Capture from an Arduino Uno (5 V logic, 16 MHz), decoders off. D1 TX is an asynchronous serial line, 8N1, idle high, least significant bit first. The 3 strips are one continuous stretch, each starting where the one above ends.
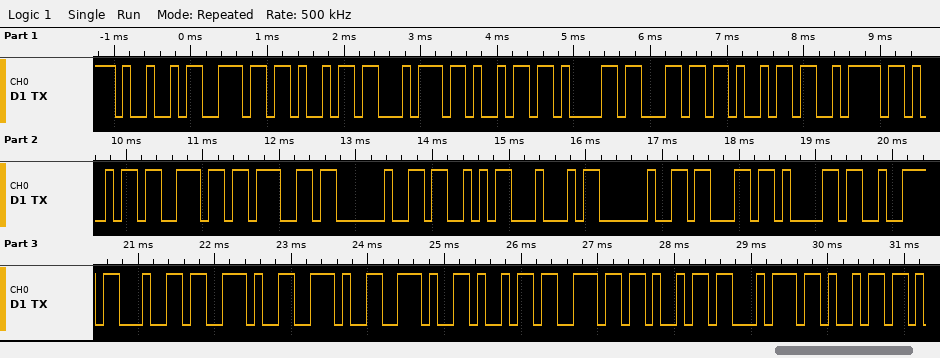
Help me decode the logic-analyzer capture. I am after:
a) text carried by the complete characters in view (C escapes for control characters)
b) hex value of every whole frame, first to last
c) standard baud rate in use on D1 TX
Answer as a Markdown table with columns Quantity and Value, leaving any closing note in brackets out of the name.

| Quantity | Value |
|---|---|
| text carried by the complete characters in view | "Initializing SD card...initi" |
| hex value of every whole frame, first to last | 49 6E 69 74 69 61 6C 69 7A 69 6E 67 20 53 44 20 63 61 72 64 2E 2E 2E 69 6E 69 74 69 |
| standard baud rate in use on D1 TX | 9600 baud |
